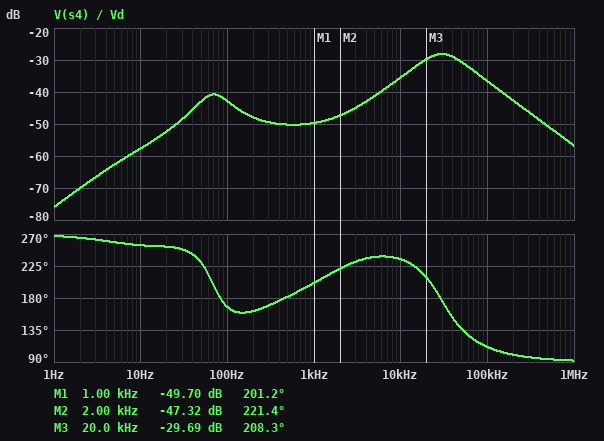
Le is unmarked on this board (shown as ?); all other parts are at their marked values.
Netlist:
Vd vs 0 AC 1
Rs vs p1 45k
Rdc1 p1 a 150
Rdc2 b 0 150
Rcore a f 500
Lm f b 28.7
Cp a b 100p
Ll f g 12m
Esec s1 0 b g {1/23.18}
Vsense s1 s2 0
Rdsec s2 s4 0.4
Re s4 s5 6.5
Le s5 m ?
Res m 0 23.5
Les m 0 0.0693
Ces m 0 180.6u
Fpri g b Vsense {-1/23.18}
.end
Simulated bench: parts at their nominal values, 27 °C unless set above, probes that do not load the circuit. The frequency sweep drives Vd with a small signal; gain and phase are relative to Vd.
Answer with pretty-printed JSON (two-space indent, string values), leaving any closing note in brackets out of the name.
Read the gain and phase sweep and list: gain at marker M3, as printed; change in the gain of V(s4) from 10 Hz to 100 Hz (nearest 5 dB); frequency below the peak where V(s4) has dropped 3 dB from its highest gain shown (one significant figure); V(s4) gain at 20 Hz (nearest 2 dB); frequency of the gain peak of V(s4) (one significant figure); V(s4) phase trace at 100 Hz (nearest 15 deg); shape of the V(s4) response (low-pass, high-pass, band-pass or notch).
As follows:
{
  "gain at marker M3, as printed": "-29.69 dB",
  "change in the gain of V(s4) from 10 Hz to 100 Hz": "15 dB",
  "frequency below the peak where V(s4) has dropped 3 dB from its highest gain shown": "20 kHz",
  "V(s4) gain at 20 Hz": "-52 dB",
  "frequency of the gain peak of V(s4)": "30 kHz",
  "V(s4) phase trace at 100 Hz": "165 deg",
  "shape of the V(s4) response": "band-pass"
}
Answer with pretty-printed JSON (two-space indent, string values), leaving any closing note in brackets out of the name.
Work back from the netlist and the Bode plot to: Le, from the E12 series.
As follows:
{
  "Le, from the E12 series": "560 µH"
}
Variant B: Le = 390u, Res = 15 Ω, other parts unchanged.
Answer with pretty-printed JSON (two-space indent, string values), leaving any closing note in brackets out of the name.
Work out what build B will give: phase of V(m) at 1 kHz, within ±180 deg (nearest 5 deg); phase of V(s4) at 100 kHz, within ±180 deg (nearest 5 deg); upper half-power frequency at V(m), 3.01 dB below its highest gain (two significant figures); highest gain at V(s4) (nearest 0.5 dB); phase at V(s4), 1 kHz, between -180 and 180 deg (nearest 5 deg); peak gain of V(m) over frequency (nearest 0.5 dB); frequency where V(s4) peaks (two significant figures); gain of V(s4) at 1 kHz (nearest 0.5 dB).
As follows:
{
  "phase of V(m) at 1 kHz, within ±180 deg": "95 deg",
  "phase of V(s4) at 100 kHz, within ±180 deg": "110 deg",
  "upper half-power frequency at V(m), 3.01 dB below its highest gain": "120 Hz",
  "highest gain at V(s4)": "-28.5 dB",
  "phase at V(s4), 1 kHz, between -180 and 180 deg": "-165 deg",
  "peak gain of V(m) over frequency": "-46.0 dB",
  "frequency where V(s4) peaks": "35 kHz",
  "gain of V(s4) at 1 kHz": "-50.0 dB"
}
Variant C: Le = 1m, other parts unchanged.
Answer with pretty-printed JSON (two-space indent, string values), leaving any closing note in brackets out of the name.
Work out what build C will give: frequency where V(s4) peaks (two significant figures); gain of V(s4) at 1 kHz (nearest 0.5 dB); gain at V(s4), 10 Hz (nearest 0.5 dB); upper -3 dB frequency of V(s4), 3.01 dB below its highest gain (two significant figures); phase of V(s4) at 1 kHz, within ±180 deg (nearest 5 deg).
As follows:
{
  "frequency where V(s4) peaks": "23 kHz",
  "gain of V(s4) at 1 kHz": "-48.0 dB",
  "gain at V(s4), 10 Hz": "-57.5 dB",
  "upper -3 dB frequency of V(s4), 3.01 dB below its highest gain": "47 kHz",
  "phase of V(s4) at 1 kHz, within ±180 deg": "-145 deg"
}
